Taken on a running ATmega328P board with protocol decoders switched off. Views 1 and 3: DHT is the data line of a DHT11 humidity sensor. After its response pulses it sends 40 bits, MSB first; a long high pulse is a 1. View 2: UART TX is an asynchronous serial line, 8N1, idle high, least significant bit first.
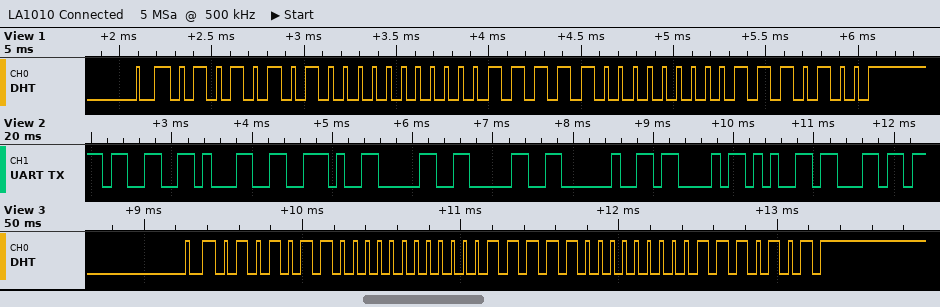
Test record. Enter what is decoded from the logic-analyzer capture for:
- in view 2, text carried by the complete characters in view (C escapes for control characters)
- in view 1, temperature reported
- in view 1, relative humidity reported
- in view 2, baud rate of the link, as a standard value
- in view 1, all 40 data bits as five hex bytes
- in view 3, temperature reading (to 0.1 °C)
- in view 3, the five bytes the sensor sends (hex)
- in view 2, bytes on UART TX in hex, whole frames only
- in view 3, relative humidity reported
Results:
"31.00 Cel"
31.0 °C
85 %
9600 baud
55 00 1F 00 74
31.0 °C
56 00 1F 00 75
33 31 2E 30 30 20 43 65 6C
86 %
